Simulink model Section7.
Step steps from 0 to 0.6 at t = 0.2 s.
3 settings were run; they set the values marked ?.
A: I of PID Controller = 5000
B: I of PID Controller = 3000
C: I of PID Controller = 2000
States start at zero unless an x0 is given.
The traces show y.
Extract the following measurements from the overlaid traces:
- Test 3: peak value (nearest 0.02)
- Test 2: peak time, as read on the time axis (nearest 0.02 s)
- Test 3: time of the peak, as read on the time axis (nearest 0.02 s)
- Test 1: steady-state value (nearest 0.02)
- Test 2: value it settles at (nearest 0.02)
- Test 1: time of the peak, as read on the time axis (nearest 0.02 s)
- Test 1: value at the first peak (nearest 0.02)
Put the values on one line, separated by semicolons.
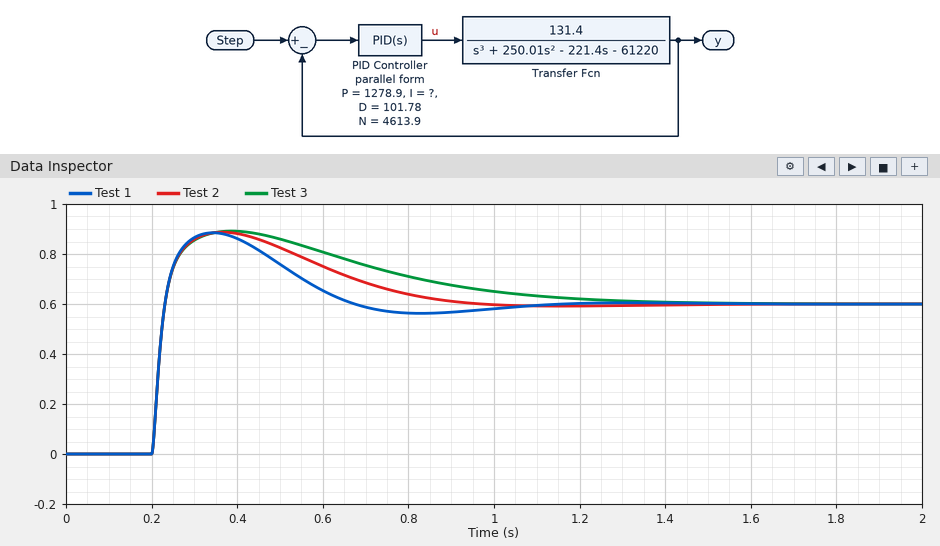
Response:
0.90; 0.36 s; 0.38 s; 0.60; 0.60; 0.34 s; 0.88
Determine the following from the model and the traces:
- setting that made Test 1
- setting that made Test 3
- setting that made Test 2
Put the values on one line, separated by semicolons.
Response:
A; C; B
